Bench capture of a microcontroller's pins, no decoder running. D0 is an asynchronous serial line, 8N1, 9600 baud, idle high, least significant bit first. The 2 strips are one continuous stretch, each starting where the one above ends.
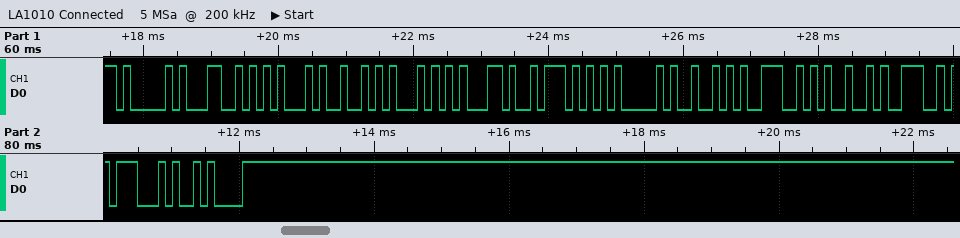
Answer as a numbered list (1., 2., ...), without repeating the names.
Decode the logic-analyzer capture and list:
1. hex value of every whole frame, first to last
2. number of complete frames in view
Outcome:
1. 0x41 0x4C 0x45 0x52 0x54 0x2C 0x57 0x41 0x52 0x4E 0x49 0x4E 0x47 0x0A
2. 14
